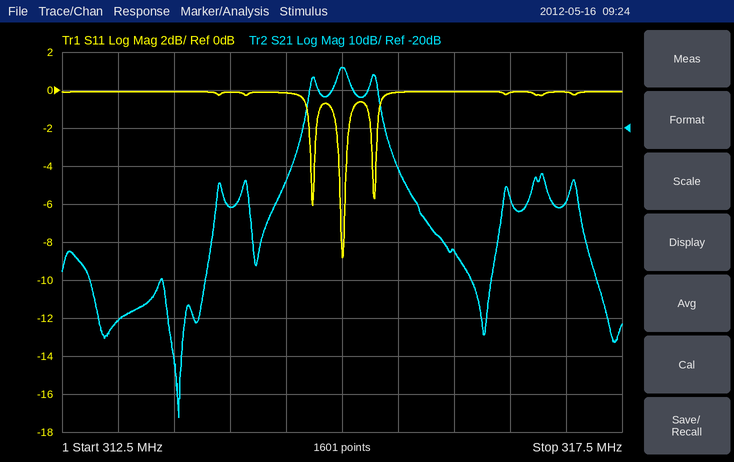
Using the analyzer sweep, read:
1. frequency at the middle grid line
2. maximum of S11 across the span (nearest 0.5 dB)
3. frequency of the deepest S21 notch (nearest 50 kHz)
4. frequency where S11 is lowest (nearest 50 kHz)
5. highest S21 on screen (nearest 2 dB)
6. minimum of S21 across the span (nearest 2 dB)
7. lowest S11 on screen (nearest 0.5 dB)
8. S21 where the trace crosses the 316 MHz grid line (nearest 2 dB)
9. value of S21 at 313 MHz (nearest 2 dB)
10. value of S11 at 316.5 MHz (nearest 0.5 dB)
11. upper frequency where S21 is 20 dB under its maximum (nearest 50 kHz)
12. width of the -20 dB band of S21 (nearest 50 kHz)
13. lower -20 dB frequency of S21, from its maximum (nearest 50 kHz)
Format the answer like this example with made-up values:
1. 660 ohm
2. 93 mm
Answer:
1. 315 MHz
2. 0.0 dB
3. 313.55 MHz
4. 315.00 MHz
5. -4 dB
6. -96 dB
7. -9.0 dB
8. -52 dB
9. -70 dB
10. 0.0 dB
11. 315.40 MHz
12. 800 kHz
13. 314.60 MHz
